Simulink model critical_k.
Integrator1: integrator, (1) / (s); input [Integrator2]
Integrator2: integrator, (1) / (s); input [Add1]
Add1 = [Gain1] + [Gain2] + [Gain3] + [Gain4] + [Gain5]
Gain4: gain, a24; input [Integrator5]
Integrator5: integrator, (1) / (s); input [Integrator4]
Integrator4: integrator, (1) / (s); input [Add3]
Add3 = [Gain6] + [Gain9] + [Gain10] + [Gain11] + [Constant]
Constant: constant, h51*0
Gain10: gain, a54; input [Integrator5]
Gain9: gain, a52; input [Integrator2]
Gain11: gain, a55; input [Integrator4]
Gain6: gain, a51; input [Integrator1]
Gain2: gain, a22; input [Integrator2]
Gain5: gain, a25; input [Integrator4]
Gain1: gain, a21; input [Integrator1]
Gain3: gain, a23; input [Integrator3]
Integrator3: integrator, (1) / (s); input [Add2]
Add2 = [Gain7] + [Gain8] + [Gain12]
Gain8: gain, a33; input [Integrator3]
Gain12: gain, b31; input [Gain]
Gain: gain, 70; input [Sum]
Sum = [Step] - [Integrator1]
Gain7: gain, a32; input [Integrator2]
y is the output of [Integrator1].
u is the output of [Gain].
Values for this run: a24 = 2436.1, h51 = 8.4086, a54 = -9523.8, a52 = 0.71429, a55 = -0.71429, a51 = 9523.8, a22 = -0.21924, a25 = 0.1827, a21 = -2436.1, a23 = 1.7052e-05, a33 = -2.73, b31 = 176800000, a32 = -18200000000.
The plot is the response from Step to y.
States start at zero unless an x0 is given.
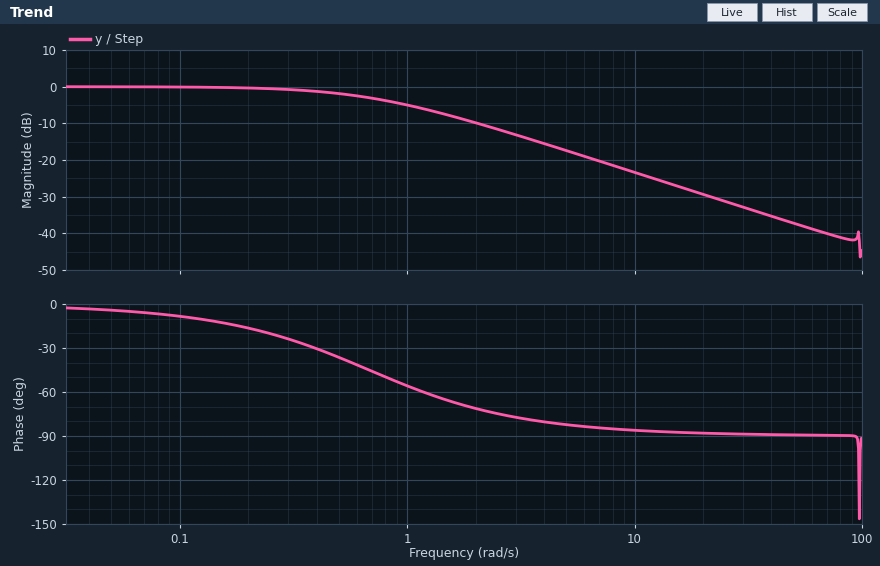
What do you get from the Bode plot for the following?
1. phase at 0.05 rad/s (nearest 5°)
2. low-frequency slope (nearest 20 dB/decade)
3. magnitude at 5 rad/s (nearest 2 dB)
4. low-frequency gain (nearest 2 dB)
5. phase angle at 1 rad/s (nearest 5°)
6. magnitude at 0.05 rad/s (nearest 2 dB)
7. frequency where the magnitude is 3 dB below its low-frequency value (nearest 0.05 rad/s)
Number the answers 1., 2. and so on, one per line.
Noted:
1. -5°
2. 0 dB/decade
3. -18 dB
4. 0 dB
5. -55°
6. 0 dB
7. 0.70 rad/s
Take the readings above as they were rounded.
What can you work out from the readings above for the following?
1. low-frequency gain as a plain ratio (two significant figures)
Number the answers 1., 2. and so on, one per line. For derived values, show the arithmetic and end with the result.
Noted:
1. 10^(0 / 20) = 1.0
